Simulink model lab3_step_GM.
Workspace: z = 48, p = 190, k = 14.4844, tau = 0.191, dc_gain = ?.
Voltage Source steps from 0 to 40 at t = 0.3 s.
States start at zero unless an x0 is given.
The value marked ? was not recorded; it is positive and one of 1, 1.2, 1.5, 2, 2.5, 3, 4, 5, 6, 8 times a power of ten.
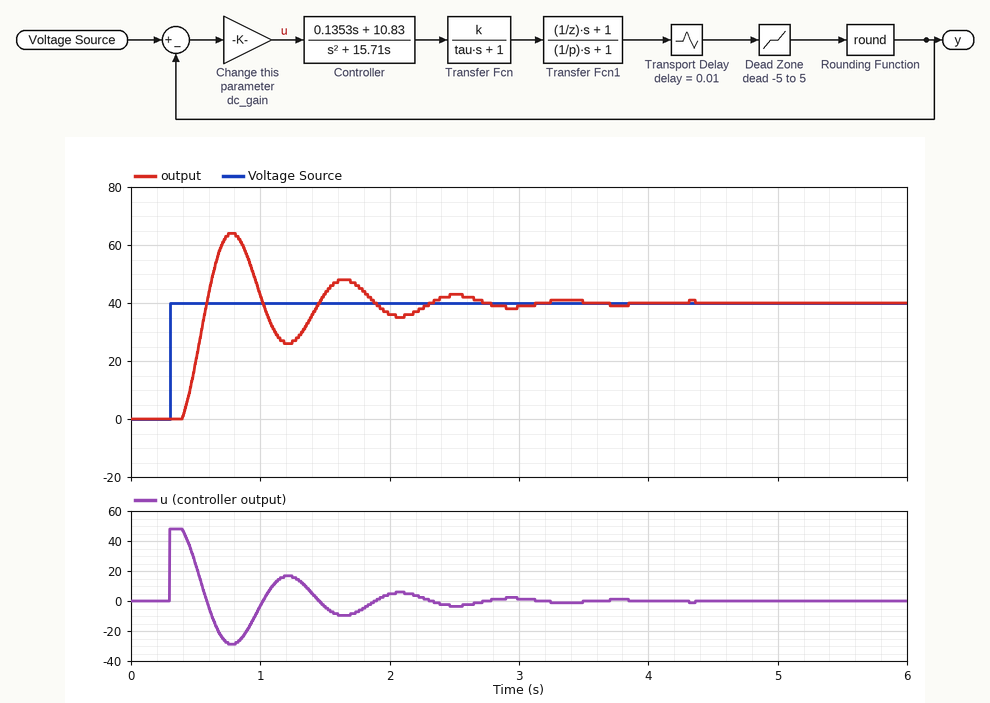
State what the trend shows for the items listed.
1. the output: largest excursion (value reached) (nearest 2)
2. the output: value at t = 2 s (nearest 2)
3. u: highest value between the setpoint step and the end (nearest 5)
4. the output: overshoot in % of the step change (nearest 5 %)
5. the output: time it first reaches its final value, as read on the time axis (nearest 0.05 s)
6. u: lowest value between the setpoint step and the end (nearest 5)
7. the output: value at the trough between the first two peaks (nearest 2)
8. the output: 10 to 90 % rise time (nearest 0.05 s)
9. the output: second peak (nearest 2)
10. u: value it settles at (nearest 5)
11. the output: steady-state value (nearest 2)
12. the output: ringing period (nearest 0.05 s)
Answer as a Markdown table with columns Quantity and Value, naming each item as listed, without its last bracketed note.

| Quantity | Value |
|---|---|
| the output: largest excursion (value reached) | 64 |
| the output: value at t = 2 s | 36 |
| u: highest value between the setpoint step and the end | 50 |
| the output: overshoot in % of the step change | 60 % |
| the output: time it first reaches its final value, as read on the time axis | 0.60 s |
| u: lowest value between the setpoint step and the end | -30 |
| the output: value at the trough between the first two peaks | 26 |
| the output: 10 to 90 % rise time | 0.15 s |
| the output: second peak | 48 |
| u: value it settles at | 0 |
| the output: steady-state value | 40 |
| the output: ringing period | 0.85 s |
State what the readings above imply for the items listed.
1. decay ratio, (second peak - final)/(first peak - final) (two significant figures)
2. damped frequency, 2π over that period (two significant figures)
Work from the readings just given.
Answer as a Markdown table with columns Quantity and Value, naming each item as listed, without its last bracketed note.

| Quantity | Value |
|---|---|
| decay ratio, (second peak - final)/(first peak - final) | 0.33 |
| damped frequency, 2π over that period | 7.4 rad/s |
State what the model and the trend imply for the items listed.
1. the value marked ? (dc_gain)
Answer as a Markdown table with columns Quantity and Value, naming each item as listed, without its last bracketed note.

| Quantity | Value |
|---|---|
| the value marked ? | 1.2 |
